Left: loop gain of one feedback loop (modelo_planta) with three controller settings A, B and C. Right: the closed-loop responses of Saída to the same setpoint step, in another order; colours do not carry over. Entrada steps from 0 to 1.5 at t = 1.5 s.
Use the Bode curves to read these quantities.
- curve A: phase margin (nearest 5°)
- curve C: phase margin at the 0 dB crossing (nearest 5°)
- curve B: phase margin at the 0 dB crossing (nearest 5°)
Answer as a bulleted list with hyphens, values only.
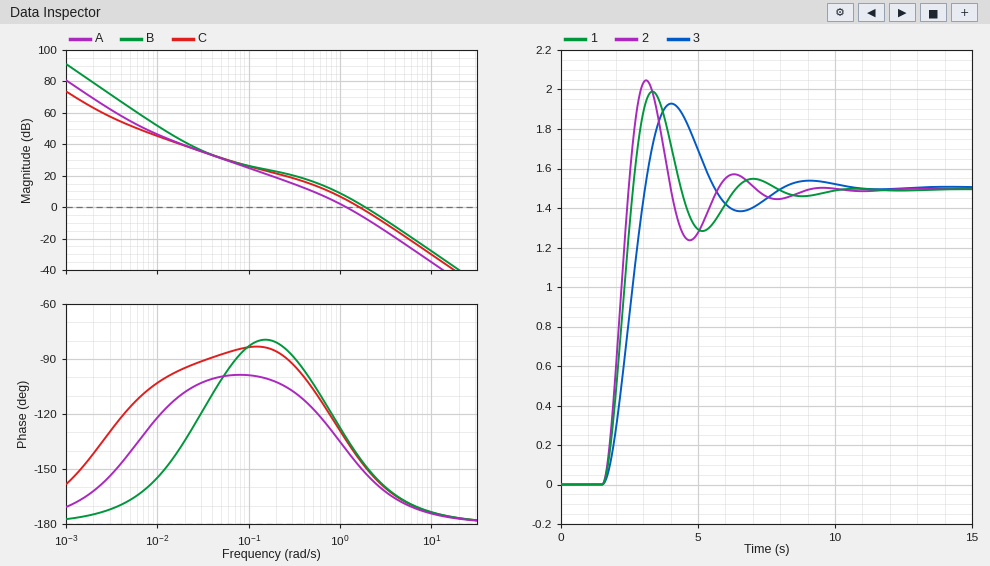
- 40°
- 35°
- 30°
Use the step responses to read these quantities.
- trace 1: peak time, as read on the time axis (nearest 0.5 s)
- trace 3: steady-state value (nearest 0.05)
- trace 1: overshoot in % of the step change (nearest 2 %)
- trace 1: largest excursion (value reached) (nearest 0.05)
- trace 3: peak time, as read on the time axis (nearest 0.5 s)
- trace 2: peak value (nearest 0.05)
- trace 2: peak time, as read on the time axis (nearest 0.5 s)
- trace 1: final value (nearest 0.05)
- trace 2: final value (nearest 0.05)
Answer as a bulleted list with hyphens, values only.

- 3.5 s
- 1.50
- 32 %
- 2.00
- 4.0 s
- 2.05
- 3.0 s
- 1.50
- 1.50
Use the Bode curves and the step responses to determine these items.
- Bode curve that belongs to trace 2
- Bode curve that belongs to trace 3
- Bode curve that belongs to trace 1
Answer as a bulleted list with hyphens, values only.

- B
- A
- C
